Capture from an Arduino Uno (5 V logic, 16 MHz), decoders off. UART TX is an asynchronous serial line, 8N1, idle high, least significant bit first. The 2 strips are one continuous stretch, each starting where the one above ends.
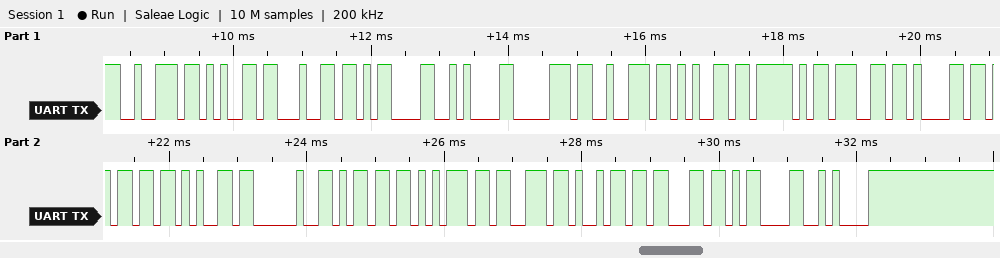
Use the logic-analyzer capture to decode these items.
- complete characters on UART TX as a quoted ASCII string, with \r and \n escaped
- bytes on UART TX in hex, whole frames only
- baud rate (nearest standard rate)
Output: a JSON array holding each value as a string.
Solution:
["\"red\\r\\npre_game music\\r\\n\"", "72 65 64 0D 0A 70 72 65 5F 67 61 6D 65 20 6D 75 73 69 63 0D 0A", "9600 baud"]
